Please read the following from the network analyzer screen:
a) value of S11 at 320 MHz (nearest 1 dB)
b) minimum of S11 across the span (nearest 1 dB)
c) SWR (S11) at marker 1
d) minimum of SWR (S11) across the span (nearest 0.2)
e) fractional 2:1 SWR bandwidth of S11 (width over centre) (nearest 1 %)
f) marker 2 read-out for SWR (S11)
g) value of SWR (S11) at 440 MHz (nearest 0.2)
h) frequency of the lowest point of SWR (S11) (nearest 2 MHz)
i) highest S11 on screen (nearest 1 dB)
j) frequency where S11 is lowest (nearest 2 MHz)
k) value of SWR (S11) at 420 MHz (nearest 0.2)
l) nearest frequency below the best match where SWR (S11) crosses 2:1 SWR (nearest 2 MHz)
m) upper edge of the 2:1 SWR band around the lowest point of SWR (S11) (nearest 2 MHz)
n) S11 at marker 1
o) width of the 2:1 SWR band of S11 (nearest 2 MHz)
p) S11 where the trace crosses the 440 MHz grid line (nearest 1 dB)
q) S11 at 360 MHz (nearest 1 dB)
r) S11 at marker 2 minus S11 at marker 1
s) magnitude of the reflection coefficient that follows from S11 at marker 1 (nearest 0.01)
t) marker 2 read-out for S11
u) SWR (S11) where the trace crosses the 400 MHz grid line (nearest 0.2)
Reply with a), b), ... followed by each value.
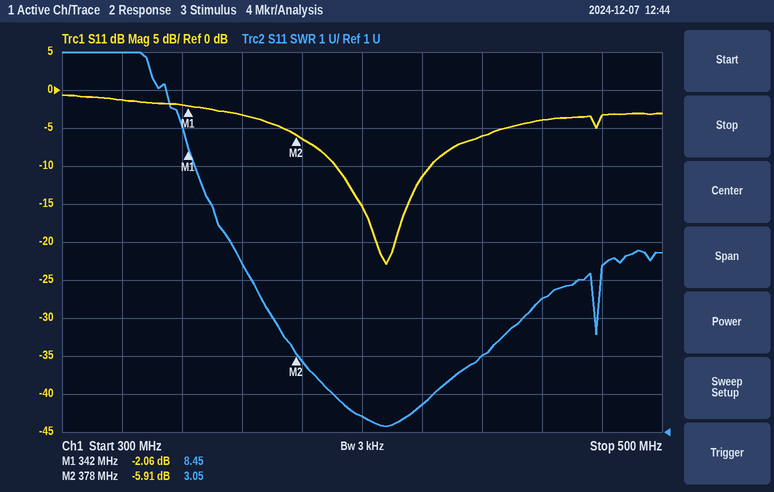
a) -1 dB
b) -23 dB
c) 8.45
d) 1.2
e) 8 %
f) 3.05
g) 3.0
h) 408 MHz
i) -1 dB
j) 408 MHz
k) 1.8
l) 390 MHz
m) 424 MHz
n) -2.06 dB
o) 34 MHz
p) -6 dB
q) -3 dB
r) -3.85 dB
s) 0.79
t) -5.91 dB
u) 1.4
